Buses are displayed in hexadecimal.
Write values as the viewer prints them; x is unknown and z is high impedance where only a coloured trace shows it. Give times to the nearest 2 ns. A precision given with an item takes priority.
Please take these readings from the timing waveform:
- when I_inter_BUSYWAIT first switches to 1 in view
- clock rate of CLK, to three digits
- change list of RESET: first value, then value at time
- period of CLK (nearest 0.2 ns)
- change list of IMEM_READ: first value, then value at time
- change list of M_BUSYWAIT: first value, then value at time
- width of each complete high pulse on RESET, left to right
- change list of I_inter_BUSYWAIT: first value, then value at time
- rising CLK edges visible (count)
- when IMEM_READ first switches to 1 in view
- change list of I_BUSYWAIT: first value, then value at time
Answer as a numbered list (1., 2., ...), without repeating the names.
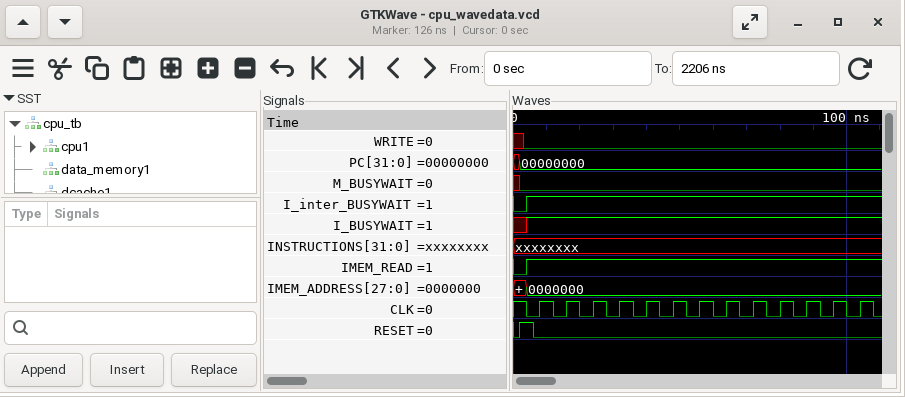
1. 4 ns
2. 125 MHz
3. 0, 1 at 2 ns, 0 at 6 ns
4. 8 ns
5. 0, 1 at 4 ns
6. x, 0 at 2 ns
7. 4 ns
8. 0, 1 at 4 ns
9. 13
10. 4 ns
11. x, 1 at 4 ns
